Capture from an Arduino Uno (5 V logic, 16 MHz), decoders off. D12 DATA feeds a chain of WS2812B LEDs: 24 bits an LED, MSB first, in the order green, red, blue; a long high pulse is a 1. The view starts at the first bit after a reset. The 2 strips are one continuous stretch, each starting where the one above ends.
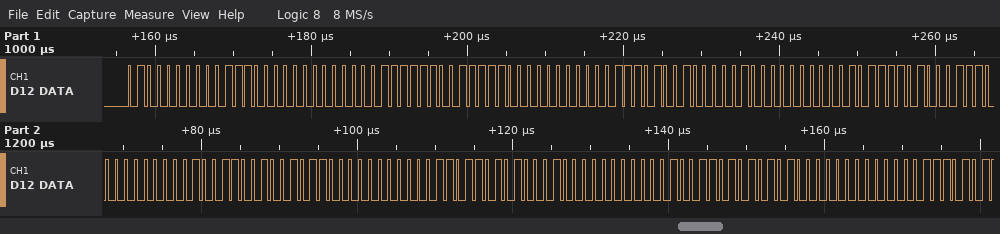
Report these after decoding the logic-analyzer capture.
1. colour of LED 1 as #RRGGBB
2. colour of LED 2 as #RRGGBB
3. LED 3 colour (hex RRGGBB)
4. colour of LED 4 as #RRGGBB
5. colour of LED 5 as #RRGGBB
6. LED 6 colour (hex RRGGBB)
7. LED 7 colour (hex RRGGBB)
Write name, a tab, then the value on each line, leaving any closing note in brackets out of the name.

colour of LED 1 as #RRGGBB	#384000
colour of LED 2 as #RRGGBB	#3E3F00
LED 3 colour	#413A00
colour of LED 4 as #RRGGBB	#472F00
colour of LED 5 as #RRGGBB	#4B2600
LED 6 colour	#511B00
LED 7 colour	#551300
